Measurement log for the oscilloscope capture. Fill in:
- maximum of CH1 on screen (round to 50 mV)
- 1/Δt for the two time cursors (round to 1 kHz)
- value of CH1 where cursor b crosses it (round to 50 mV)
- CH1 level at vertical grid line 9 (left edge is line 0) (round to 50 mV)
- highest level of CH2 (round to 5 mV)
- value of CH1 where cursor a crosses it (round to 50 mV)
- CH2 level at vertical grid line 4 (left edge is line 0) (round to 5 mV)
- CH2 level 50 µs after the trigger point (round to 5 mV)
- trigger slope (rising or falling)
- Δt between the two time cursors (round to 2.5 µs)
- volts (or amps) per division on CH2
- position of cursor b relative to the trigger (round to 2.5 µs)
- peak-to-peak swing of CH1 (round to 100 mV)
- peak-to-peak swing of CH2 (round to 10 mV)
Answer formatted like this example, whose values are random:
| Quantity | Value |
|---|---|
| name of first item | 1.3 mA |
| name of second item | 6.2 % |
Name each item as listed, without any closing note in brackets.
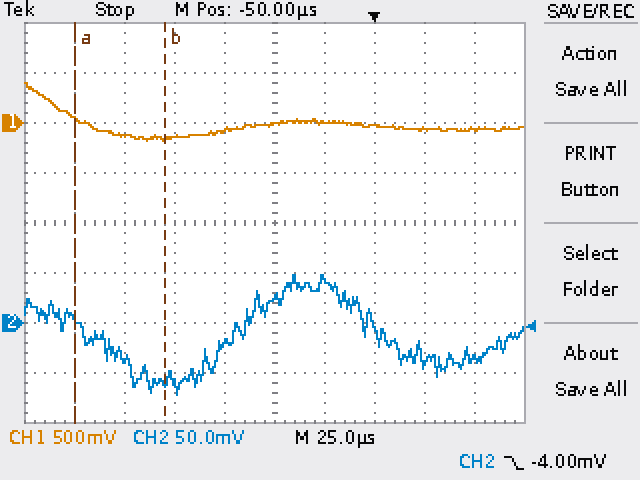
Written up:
| Quantity | Value |
|---|---|
| maximum of CH1 on screen | 400 mV |
| 1/Δt for the two time cursors | 22 kHz |
| value of CH1 where cursor b crosses it | -150 mV |
| CH1 level at vertical grid line 9 (left edge is line 0) | -50 mV |
| highest level of CH2 | 50 mV |
| value of CH1 where cursor a crosses it | 50 mV |
| CH2 level at vertical grid line 4 (left edge is line 0) | -20 mV |
| CH2 level 50 µs after the trigger point | -35 mV |
| trigger slope | falling |
| Δt between the two time cursors | 45.0 µs |
| volts (or amps) per division on CH2 | 50 mV |
| position of cursor b relative to the trigger | -105.0 µs |
| peak-to-peak swing of CH1 | 600 mV |
| peak-to-peak swing of CH2 | 120 mV |
